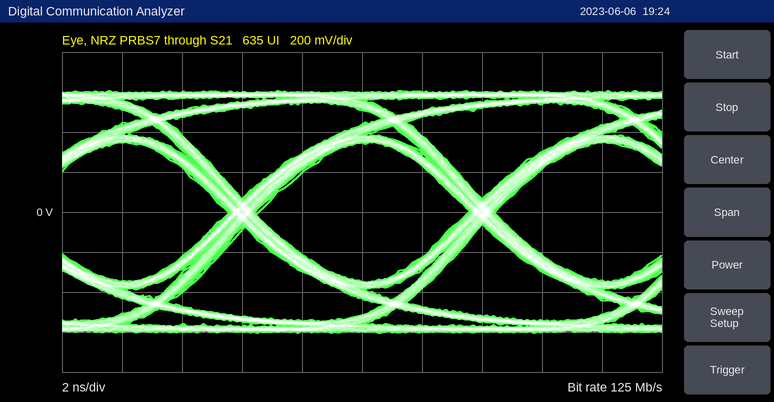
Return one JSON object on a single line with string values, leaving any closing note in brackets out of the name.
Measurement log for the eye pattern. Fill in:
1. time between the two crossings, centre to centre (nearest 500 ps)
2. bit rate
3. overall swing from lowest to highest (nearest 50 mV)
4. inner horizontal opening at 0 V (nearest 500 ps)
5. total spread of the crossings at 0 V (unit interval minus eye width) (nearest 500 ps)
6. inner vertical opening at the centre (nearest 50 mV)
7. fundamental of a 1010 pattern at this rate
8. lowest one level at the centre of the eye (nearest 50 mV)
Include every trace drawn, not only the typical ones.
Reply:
{"time between the two crossings, centre to centre": "8.0 ns", "bit rate": "125 Mb/s", "overall swing from lowest to highest": "1.20 V", "inner horizontal opening at 0 V": "7.0 ns", "total spread of the crossings at 0 V (unit interval minus eye width)": "1.0 ns", "inner vertical opening at the centre": "700 mV", "fundamental of a 1010 pattern at this rate": "62.5 MHz", "lowest one level at the centre of the eye": "350 mV"}
